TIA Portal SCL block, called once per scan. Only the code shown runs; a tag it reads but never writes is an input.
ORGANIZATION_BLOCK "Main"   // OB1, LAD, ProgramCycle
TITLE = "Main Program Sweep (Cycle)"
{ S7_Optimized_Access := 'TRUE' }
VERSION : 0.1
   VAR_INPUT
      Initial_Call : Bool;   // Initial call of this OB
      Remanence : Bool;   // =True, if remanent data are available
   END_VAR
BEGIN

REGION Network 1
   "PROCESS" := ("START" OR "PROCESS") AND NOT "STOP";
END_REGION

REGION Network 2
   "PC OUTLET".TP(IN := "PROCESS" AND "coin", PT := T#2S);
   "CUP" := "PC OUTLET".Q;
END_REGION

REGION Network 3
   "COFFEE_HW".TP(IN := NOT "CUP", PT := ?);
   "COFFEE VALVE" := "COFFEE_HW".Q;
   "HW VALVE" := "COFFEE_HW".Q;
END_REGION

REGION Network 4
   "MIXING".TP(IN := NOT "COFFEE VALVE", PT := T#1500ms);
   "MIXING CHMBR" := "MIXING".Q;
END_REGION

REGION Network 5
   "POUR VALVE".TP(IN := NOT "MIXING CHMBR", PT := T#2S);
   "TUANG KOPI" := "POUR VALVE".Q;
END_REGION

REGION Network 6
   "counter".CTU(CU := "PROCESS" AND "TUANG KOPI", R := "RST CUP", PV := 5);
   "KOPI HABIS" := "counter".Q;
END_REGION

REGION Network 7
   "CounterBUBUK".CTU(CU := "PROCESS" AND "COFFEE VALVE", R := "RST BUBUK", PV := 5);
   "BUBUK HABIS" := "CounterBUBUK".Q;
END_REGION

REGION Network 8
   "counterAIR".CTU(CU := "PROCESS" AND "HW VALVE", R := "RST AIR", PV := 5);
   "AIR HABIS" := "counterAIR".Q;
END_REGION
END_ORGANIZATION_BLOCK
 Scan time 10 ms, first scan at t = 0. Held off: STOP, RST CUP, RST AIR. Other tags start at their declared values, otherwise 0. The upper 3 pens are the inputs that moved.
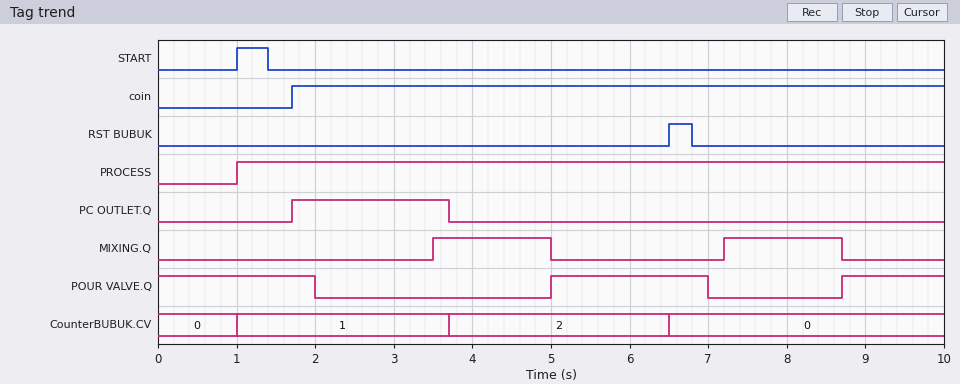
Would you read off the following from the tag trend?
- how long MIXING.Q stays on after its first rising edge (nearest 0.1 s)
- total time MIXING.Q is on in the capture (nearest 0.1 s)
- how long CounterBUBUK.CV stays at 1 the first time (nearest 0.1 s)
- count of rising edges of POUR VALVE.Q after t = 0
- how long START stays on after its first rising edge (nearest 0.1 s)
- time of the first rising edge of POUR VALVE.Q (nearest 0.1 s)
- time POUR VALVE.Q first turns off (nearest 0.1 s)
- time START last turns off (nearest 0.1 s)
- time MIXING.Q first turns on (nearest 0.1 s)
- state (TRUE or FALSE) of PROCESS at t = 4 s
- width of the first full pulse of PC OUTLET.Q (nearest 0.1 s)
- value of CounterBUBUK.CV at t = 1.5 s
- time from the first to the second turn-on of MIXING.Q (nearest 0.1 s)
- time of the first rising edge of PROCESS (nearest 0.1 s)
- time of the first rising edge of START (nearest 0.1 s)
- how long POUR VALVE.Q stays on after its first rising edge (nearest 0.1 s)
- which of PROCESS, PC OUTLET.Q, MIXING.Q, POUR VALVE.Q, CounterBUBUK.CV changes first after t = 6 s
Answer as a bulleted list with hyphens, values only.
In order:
- 1.5 s
- 3.0 s
- 2.7 s
- 2
- 0.4 s
- 5.0 s
- 2.0 s
- 1.4 s
- 3.5 s
- TRUE
- 2.0 s
- 1
- 3.7 s
- 1.0 s
- 1.0 s
- 2.0 s
- CounterBUBUK.CV
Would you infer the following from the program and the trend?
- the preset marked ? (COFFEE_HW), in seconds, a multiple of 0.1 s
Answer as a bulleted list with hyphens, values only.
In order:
- 3.5 s
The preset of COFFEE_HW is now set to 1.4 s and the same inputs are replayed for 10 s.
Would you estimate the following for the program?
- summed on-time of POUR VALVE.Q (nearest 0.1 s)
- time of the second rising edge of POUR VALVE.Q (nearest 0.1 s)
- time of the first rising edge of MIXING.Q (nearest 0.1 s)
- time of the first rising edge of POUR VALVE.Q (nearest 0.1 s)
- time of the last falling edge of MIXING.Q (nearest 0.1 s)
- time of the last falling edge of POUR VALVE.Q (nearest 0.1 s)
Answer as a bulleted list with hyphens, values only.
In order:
- 6.0 s
- 6.6 s
- 1.4 s
- 2.9 s
- 6.6 s
- 8.6 s
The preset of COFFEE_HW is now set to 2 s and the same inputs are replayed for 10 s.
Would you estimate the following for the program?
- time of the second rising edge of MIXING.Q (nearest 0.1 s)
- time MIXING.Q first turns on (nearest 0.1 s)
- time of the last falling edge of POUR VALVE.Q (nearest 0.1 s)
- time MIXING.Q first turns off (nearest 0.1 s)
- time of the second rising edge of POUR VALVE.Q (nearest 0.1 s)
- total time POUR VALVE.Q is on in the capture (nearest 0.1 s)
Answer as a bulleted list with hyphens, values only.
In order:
- 5.7 s
- 2.0 s
- 9.2 s
- 3.5 s
- 7.2 s
- 6.0 s
